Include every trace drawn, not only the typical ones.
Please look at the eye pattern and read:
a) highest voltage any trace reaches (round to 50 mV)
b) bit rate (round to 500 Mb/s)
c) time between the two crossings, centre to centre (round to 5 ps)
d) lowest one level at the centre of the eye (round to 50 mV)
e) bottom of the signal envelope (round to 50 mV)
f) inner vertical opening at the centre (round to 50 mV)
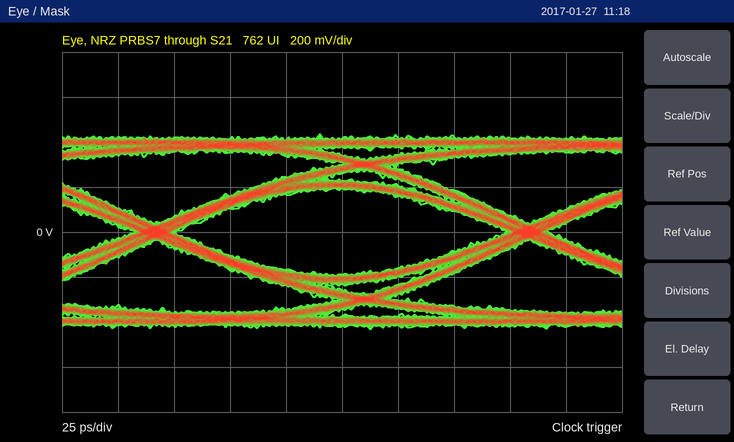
450 mV
6.0 Gb/s
165 ps
200 mV
-450 mV
400 mV
